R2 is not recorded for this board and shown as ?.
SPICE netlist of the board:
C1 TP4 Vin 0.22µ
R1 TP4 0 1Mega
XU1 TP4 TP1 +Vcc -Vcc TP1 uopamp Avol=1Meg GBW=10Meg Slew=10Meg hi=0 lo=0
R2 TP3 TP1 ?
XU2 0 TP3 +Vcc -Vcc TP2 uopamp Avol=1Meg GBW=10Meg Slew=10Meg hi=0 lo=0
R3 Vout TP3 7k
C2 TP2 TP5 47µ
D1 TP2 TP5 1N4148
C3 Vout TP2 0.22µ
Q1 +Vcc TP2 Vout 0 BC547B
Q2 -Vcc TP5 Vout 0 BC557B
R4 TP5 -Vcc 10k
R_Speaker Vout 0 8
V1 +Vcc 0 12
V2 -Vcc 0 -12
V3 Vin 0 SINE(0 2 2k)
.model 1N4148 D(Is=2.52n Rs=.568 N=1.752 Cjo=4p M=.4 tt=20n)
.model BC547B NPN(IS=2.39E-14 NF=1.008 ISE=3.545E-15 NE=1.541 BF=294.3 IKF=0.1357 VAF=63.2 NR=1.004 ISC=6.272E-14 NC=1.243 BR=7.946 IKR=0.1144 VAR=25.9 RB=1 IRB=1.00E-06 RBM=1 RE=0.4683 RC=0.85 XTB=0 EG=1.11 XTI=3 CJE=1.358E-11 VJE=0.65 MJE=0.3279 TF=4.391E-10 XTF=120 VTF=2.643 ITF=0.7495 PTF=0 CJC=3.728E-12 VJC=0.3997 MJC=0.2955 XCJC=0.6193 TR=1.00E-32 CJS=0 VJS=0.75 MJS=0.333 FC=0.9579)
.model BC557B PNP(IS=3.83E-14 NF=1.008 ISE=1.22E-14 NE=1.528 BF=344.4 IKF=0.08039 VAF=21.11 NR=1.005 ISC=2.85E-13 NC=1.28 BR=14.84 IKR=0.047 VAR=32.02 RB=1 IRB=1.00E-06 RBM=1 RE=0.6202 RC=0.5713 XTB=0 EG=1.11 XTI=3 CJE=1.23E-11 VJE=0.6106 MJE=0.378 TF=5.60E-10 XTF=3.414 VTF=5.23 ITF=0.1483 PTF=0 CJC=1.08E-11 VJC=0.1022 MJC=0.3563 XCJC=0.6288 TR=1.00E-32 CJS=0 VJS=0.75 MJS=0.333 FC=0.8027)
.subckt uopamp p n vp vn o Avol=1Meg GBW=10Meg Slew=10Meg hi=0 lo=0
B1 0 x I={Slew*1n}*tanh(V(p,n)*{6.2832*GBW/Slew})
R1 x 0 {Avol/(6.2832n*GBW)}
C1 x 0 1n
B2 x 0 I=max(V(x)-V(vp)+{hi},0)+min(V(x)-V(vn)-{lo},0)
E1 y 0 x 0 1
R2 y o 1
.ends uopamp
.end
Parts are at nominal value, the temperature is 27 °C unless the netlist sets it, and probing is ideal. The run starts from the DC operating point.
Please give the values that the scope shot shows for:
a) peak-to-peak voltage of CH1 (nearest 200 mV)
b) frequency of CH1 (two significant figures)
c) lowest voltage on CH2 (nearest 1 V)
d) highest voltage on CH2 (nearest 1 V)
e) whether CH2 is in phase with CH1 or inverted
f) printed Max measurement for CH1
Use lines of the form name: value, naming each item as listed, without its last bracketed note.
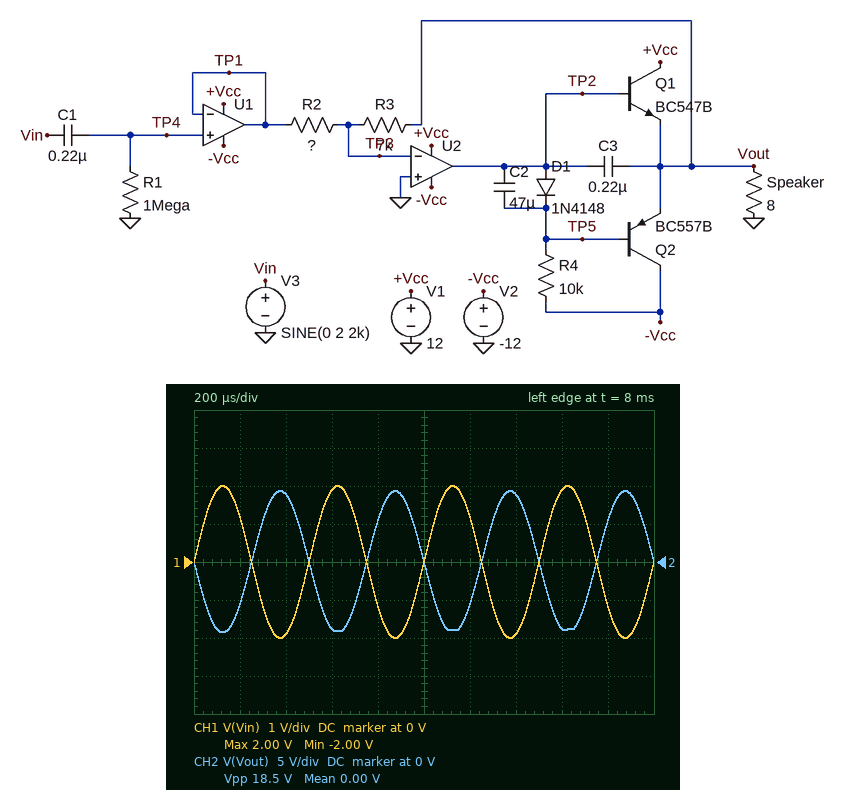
peak-to-peak voltage of CH1: 4.0 V
frequency of CH1: 2.0 kHz
lowest voltage on CH2: -9 V
highest voltage on CH2: 9 V
whether CH2 is in phase with CH1 or inverted: inverted
printed Max measurement for CH1: 2.00 V
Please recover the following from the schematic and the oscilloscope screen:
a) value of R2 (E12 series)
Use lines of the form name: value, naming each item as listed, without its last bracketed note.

value of R2: 1.5 kΩ
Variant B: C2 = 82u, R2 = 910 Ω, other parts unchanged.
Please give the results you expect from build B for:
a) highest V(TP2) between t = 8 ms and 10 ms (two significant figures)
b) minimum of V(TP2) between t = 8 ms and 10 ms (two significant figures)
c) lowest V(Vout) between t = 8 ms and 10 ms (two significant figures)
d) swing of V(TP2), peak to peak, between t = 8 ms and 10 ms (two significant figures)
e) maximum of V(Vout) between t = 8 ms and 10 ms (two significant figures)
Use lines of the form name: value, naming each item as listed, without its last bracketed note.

highest V(TP2) between t = 8 ms and 10 ms: 12 V
minimum of V(TP2) between t = 8 ms and 10 ms: -12 V
lowest V(Vout) between t = 8 ms and 10 ms: -9.0 V
swing of V(TP2), peak to peak, between t = 8 ms and 10 ms: 24 V
maximum of V(Vout) between t = 8 ms and 10 ms: 10 V
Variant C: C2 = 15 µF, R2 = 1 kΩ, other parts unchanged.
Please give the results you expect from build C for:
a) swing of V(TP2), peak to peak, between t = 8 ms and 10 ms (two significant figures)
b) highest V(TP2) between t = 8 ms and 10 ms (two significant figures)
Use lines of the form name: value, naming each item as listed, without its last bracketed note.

swing of V(TP2), peak to peak, between t = 8 ms and 10 ms: 24 V
highest V(TP2) between t = 8 ms and 10 ms: 12 V
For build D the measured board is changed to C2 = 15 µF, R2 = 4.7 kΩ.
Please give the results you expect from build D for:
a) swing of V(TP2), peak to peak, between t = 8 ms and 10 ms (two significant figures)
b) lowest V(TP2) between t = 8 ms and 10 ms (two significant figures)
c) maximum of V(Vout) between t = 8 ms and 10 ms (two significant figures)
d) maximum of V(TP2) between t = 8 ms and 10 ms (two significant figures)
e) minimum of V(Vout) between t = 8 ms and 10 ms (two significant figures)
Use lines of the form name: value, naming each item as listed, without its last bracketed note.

swing of V(TP2), peak to peak, between t = 8 ms and 10 ms: 7.5 V
lowest V(TP2) between t = 8 ms and 10 ms: -3.5 V
maximum of V(Vout) between t = 8 ms and 10 ms: 3.0 V
maximum of V(TP2) between t = 8 ms and 10 ms: 4.0 V
minimum of V(Vout) between t = 8 ms and 10 ms: -3.0 V
